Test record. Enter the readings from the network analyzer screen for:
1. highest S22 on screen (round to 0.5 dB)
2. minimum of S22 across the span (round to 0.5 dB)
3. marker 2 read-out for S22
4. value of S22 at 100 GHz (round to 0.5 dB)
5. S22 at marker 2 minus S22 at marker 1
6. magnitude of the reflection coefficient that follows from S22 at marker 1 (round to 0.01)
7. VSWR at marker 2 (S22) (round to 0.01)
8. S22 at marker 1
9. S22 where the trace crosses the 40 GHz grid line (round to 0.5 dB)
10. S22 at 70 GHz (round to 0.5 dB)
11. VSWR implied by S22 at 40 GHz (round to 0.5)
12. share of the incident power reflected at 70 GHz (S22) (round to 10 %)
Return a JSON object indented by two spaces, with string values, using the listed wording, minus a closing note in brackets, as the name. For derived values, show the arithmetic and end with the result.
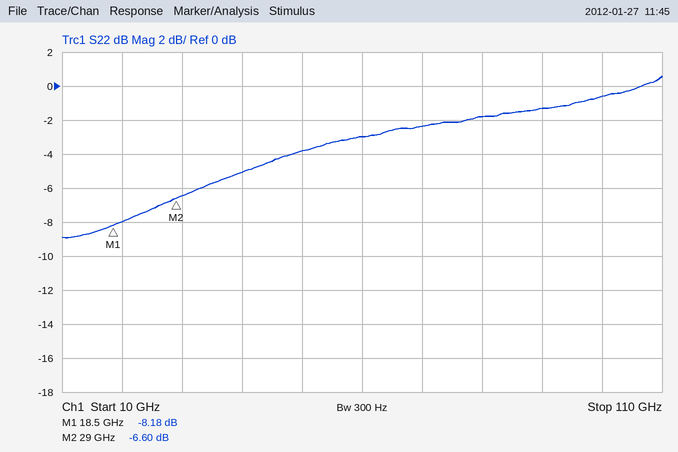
{
  "highest S22 on screen": "0.5 dB",
  "minimum of S22 across the span": "-9.0 dB",
  "marker 2 read-out for S22": "-6.60 dB",
  "value of S22 at 100 GHz": "-0.5 dB",
  "S22 at marker 2 minus S22 at marker 1": "-6.6 − (-8.18) = 1.58 dB",
  "magnitude of the reflection coefficient that follows from S22 at marker 1": "10^(-8.18/20) ≈ 0.39",
  "VSWR at marker 2 (S22)": "(1 + 0.4677)/(1 − 0.4677) ≈ 2.76",
  "S22 at marker 1": "-8.18 dB",
  "S22 where the trace crosses the 40 GHz grid line": "-5.0 dB",
  "S22 at 70 GHz": "-2.5 dB",
  "VSWR implied by S22 at 40 GHz": "|Γ| = 10^(-5/20) = 0.5623; VSWR = (1 + 0.5623)/(1 − 0.5623) ≈ 3.57, so 3.5 to the nearest 0.5",
  "share of the incident power reflected at 70 GHz (S22)": "10^(-2.5/10) ≈ 56.2 %, so 60 % to the nearest 10 %"
}
